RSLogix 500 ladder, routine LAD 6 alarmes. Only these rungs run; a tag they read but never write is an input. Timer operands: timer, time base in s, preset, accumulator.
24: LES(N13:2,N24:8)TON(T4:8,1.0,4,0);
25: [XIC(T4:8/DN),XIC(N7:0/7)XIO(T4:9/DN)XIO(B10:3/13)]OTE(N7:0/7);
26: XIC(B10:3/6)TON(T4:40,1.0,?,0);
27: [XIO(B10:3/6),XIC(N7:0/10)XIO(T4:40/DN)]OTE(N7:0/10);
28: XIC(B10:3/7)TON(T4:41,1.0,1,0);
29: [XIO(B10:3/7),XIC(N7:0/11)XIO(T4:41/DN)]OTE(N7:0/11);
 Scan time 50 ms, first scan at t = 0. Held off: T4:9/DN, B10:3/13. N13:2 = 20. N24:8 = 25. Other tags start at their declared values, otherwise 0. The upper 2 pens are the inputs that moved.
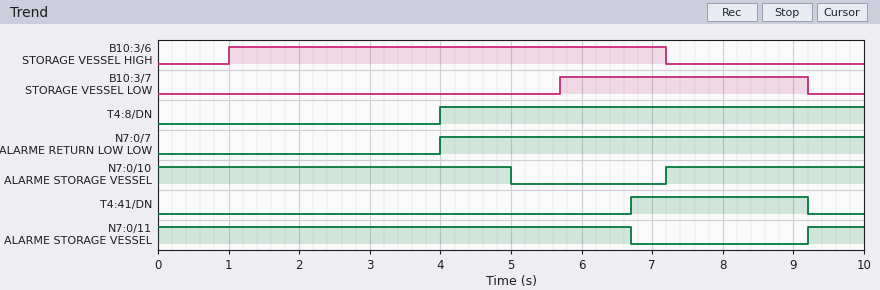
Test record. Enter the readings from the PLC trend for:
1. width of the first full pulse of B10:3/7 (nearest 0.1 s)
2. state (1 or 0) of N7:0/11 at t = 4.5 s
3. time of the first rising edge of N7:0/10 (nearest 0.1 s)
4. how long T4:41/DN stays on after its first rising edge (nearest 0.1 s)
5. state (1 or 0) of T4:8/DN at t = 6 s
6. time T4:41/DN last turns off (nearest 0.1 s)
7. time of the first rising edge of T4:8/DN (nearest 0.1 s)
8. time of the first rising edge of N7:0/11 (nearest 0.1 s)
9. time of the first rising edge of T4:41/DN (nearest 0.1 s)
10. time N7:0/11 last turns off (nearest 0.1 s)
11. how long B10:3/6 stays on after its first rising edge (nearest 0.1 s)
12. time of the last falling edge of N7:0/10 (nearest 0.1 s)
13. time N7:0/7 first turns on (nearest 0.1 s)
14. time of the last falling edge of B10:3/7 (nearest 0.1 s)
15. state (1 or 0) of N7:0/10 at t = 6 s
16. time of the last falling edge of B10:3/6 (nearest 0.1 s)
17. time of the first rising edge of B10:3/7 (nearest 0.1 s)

3.5 s
1
7.2 s
2.5 s
1
9.2 s
4.0 s
9.2 s
6.7 s
6.7 s
6.2 s
5.0 s
4.0 s
9.2 s
0
7.2 s
5.7 s
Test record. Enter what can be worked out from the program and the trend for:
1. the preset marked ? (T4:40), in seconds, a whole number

4 s
